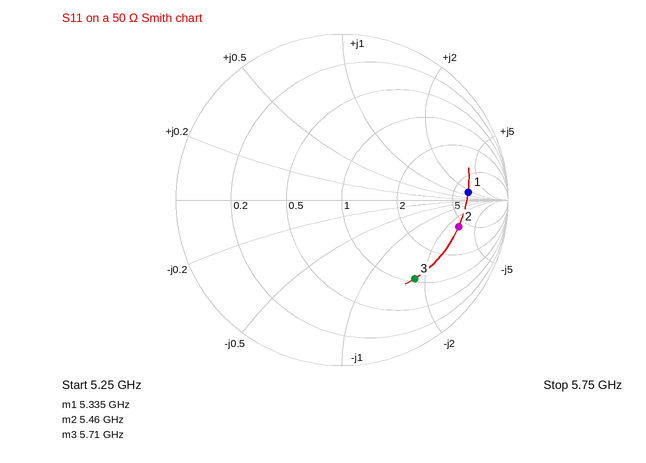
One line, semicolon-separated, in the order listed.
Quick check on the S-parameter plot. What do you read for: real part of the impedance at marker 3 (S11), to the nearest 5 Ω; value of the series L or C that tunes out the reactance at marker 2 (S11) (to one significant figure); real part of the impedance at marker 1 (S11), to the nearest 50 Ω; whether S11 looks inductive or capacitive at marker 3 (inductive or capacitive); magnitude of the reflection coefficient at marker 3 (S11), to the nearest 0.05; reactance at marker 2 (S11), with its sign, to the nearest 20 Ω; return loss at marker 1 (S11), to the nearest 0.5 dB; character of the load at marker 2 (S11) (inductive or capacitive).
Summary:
55 Ω; 4 nH; 350 Ω; capacitive; 0.65; -140 Ω; 2.5 dB; capacitive
